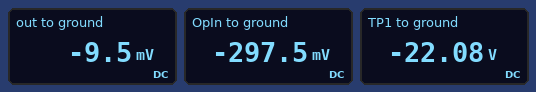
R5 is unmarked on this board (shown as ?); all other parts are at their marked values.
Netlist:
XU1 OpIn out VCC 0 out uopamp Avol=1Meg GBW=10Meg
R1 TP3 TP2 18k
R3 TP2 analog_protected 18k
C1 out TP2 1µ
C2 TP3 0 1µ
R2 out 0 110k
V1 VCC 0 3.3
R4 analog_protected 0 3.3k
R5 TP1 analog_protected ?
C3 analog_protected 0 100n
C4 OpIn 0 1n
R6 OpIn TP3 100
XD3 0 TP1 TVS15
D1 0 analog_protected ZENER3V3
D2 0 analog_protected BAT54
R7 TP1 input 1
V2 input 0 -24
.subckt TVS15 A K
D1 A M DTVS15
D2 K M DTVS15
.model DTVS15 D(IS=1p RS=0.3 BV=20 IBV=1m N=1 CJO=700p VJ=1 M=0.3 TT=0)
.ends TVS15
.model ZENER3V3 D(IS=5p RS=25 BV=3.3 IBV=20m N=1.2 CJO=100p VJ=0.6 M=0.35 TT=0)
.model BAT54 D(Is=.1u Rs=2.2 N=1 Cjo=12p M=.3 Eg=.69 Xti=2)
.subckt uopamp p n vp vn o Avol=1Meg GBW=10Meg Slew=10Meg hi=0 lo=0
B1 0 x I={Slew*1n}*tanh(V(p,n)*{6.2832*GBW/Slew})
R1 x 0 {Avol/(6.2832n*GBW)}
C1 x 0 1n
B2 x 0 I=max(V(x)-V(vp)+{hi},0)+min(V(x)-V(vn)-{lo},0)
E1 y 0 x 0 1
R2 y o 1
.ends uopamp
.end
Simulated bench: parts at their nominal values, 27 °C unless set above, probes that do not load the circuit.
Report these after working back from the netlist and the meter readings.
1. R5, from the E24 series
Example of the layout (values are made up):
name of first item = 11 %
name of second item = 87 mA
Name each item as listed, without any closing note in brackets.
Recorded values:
R5, from the E24 series = 3.6 kΩ
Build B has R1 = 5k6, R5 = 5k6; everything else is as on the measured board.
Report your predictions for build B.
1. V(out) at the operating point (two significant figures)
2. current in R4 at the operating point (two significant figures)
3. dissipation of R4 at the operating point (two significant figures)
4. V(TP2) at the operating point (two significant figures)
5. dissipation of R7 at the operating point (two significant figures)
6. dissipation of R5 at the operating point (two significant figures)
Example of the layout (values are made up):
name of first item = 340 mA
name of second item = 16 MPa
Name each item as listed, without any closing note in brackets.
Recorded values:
V(out) at the operating point = -9.4 mV
current in R4 at the operating point = 85 µA
dissipation of R4 at the operating point = 24 µW
V(TP2) at the operating point = -280 mV
dissipation of R7 at the operating point = 3.7 W
dissipation of R5 at the operating point = 85 mW
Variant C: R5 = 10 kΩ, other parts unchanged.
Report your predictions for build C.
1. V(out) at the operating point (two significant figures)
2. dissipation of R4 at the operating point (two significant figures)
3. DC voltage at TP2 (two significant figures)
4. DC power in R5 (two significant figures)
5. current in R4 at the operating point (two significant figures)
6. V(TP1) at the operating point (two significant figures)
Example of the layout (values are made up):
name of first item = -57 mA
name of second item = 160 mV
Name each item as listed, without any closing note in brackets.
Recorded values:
V(out) at the operating point = -9.2 mV
dissipation of R4 at the operating point = 21 µW
DC voltage at TP2 = -260 mV
DC power in R5 = 48 mW
current in R4 at the operating point = 79 µA
V(TP1) at the operating point = -22 V
